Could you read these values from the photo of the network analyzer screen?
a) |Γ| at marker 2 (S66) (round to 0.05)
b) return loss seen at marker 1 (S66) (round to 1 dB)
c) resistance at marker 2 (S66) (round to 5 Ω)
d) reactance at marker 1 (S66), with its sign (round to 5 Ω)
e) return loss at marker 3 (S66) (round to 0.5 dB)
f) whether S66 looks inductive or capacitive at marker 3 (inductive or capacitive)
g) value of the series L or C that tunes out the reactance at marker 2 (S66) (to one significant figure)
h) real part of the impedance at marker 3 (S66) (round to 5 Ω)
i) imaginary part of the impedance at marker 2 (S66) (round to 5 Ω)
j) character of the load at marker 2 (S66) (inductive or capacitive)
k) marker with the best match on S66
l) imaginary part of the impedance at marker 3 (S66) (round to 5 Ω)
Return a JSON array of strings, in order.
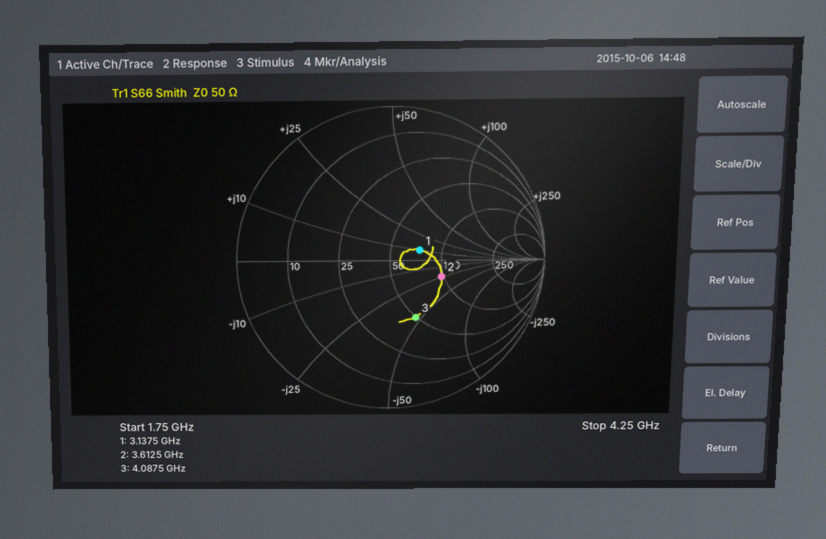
["0.35", "14 dB", "95 Ω", "+10 Ω", "7.5 dB", "capacitive", "1 nH", "50 Ω", "-25 Ω", "capacitive", "marker 1", "-45 Ω"]
